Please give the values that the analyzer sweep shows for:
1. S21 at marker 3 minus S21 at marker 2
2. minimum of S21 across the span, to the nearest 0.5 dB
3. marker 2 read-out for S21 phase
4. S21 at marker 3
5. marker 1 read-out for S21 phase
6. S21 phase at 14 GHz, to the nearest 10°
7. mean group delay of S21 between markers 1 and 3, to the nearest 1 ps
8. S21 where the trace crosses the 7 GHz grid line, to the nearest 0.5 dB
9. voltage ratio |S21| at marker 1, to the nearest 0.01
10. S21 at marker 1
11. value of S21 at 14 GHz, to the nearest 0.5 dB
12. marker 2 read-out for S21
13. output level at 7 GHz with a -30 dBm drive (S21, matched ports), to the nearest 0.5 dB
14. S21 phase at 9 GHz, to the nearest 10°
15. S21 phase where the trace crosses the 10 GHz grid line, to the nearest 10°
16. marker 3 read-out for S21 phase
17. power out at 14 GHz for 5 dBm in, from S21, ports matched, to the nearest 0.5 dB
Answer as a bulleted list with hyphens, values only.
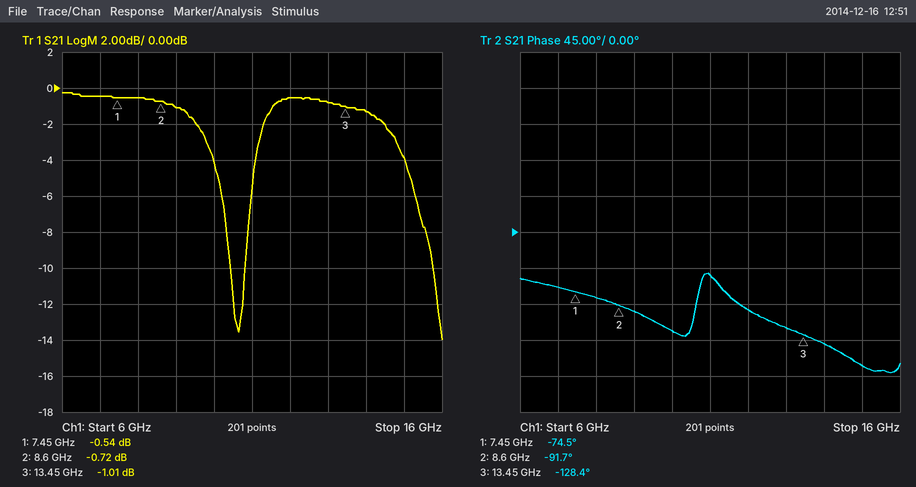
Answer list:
- -0.29 dB
- -14.0 dB
- -91.7°
- -1.01 dB
- -74.5°
- -140°
- 25 ps
- -0.5 dB
- 0.94
- -0.54 dB
- -1.5 dB
- -0.72 dB
- -30.5 dBm
- -100°
- -120°
- -128.4°
- 3.5 dBm
